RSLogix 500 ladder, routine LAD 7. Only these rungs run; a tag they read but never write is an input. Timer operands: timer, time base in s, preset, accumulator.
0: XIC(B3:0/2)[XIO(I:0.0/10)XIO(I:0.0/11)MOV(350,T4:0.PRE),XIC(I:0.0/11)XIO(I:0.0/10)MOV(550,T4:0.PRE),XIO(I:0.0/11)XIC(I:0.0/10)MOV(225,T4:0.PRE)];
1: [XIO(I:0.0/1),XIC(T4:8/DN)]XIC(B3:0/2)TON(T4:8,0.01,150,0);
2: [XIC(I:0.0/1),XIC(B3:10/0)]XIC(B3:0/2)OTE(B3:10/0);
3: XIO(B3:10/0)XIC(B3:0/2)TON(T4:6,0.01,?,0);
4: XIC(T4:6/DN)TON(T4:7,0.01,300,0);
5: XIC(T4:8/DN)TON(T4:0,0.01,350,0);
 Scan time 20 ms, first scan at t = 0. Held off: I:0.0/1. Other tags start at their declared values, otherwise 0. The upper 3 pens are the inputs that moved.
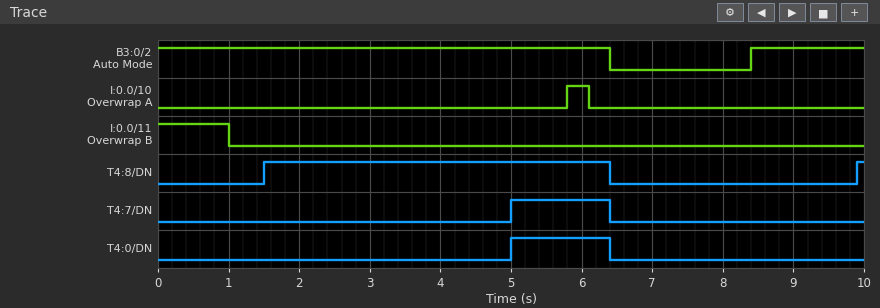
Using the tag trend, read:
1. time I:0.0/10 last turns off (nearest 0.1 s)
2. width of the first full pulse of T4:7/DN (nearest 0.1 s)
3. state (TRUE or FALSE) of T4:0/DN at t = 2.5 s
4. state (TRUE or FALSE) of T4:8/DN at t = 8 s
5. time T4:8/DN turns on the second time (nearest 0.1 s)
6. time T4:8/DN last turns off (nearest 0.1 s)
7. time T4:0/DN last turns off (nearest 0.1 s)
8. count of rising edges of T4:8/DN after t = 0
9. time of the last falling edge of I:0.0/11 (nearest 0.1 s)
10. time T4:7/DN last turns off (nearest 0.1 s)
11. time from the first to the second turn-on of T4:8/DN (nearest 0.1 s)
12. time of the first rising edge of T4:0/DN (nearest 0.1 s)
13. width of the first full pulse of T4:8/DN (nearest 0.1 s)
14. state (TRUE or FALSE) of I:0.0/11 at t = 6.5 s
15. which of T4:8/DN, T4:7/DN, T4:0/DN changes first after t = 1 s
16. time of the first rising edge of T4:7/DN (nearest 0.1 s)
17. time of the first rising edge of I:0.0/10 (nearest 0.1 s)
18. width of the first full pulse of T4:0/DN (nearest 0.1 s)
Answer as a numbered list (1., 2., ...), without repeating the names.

1. 6.1 s
2. 1.4 s
3. FALSE
4. FALSE
5. 9.9 s
6. 6.4 s
7. 6.4 s
8. 2
9. 1.0 s
10. 6.4 s
11. 8.4 s
12. 5.0 s
13. 4.9 s
14. FALSE
15. T4:8/DN
16. 5.0 s
17. 5.8 s
18. 1.4 s
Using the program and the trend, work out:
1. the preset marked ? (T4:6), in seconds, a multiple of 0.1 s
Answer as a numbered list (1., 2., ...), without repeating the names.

1. 2.0 s
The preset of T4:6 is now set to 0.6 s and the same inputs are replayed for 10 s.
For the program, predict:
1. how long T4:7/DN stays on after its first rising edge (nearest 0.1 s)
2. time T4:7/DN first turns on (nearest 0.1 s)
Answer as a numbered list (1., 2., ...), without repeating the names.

1. 2.8 s
2. 3.6 s
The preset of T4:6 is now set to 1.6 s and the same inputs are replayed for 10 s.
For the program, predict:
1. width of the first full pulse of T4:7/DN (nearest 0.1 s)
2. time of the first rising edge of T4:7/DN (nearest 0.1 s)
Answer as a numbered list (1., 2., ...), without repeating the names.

1. 1.8 s
2. 4.6 s
